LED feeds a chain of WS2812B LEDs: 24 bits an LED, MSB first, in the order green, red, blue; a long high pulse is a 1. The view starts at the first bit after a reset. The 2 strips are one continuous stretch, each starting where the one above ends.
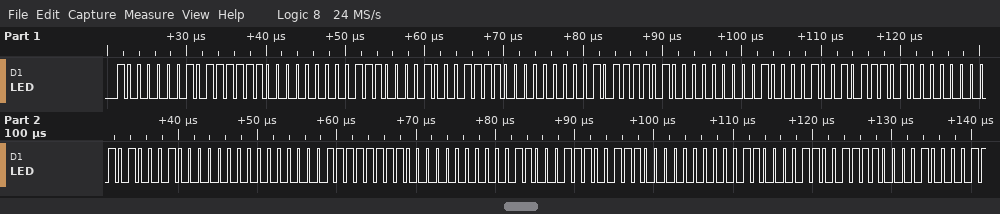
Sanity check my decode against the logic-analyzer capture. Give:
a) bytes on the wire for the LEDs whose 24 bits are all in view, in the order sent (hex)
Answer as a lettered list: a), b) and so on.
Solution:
a) 81 7E 00 E1 1E 00 BD 00 42 5D 00 A2 00 03 FC 00 63 9C 00 C3 3C
